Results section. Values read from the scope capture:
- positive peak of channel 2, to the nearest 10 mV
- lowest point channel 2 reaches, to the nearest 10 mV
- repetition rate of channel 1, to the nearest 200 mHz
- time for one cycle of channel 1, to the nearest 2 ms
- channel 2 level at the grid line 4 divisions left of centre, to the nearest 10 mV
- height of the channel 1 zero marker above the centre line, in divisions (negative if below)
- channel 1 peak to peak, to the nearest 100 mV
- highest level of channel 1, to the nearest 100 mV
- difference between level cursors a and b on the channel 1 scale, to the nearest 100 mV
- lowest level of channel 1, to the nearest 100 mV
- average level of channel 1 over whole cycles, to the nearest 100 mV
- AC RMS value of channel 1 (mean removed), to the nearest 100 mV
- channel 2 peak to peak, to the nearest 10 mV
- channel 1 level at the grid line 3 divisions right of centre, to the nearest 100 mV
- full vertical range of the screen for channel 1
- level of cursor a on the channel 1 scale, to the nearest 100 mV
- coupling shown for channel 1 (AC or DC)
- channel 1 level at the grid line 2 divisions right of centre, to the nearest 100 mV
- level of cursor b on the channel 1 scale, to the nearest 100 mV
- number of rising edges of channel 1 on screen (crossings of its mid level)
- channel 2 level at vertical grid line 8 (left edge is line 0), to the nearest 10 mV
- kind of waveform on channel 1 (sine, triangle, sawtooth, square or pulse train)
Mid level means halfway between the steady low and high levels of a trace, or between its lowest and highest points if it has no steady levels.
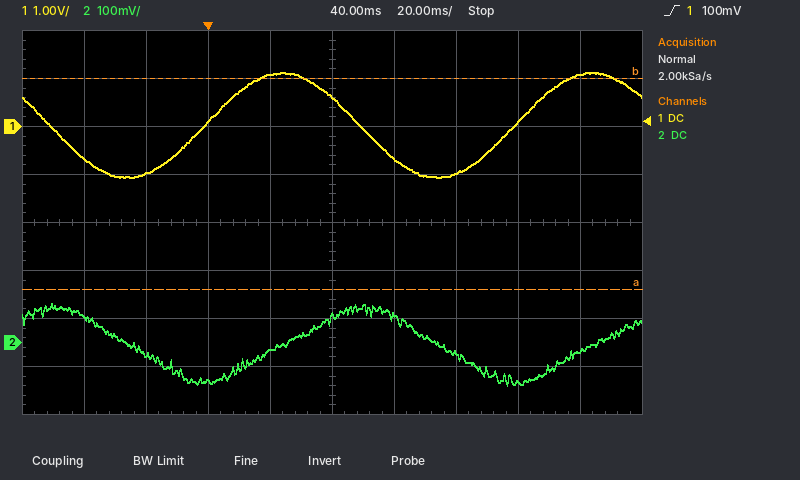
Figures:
80 mV
-90 mV
10.0 Hz
100 ms
50 mV
+2.0 div
2.2 V
1.1 V
4.4 V
-1.1 V
0.0 V
800 mV
170 mV
100 mV
8 V
-3.4 V
DC
-1.0 V
1.0 V
2
-80 mV
sine
